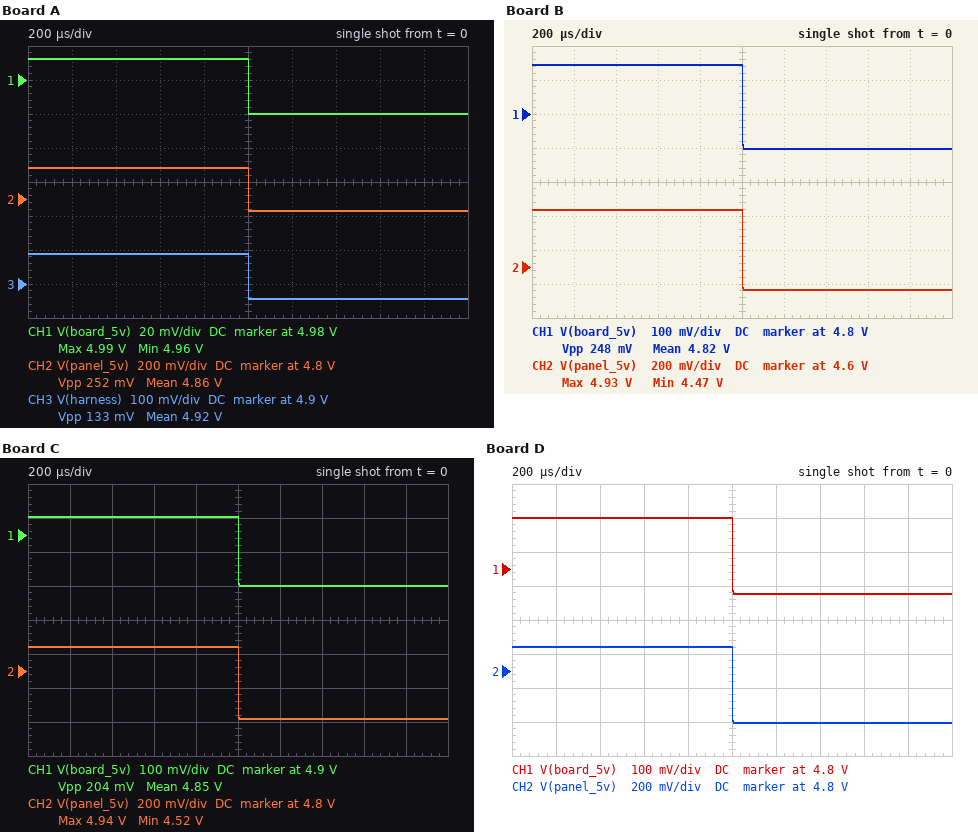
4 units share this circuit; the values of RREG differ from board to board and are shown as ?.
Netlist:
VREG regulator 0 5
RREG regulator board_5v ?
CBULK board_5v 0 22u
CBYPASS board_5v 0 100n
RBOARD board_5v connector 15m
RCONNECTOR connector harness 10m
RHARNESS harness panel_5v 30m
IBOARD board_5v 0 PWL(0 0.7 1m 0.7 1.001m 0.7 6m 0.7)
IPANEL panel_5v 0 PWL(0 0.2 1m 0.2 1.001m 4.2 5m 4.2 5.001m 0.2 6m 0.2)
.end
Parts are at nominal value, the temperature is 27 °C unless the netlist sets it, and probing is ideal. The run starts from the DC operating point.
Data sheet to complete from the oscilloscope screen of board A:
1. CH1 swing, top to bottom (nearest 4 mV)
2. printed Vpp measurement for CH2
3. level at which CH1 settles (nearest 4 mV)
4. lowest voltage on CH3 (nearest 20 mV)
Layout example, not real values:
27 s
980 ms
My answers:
32 mV
252 mV
4.960 V
4.86 V
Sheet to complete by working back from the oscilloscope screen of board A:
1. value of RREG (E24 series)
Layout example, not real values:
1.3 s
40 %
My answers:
8.2 mΩ
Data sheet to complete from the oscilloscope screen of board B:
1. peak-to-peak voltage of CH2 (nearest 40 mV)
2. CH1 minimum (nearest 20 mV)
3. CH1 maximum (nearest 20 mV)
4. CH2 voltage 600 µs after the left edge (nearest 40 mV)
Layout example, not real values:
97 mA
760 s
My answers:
480 mV
4.70 V
4.94 V
4.92 V
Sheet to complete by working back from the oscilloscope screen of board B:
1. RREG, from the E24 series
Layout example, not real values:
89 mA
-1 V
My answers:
0.062 Ω
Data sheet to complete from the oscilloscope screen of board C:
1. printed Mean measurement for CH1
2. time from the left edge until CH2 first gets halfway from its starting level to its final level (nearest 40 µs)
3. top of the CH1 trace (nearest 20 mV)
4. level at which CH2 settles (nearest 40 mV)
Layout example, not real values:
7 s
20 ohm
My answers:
4.85 V
1.00 ms
4.96 V
4.52 V
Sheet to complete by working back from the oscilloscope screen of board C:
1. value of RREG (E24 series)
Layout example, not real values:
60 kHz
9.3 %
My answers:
0.051 Ω
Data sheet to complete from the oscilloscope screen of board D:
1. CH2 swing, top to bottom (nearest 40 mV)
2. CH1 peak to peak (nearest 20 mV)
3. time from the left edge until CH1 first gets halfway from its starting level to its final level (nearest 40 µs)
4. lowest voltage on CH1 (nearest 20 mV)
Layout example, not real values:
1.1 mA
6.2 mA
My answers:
440 mV
220 mV
1.00 ms
4.72 V
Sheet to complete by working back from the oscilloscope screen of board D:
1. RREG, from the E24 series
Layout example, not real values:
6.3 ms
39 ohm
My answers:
0.056 Ω
